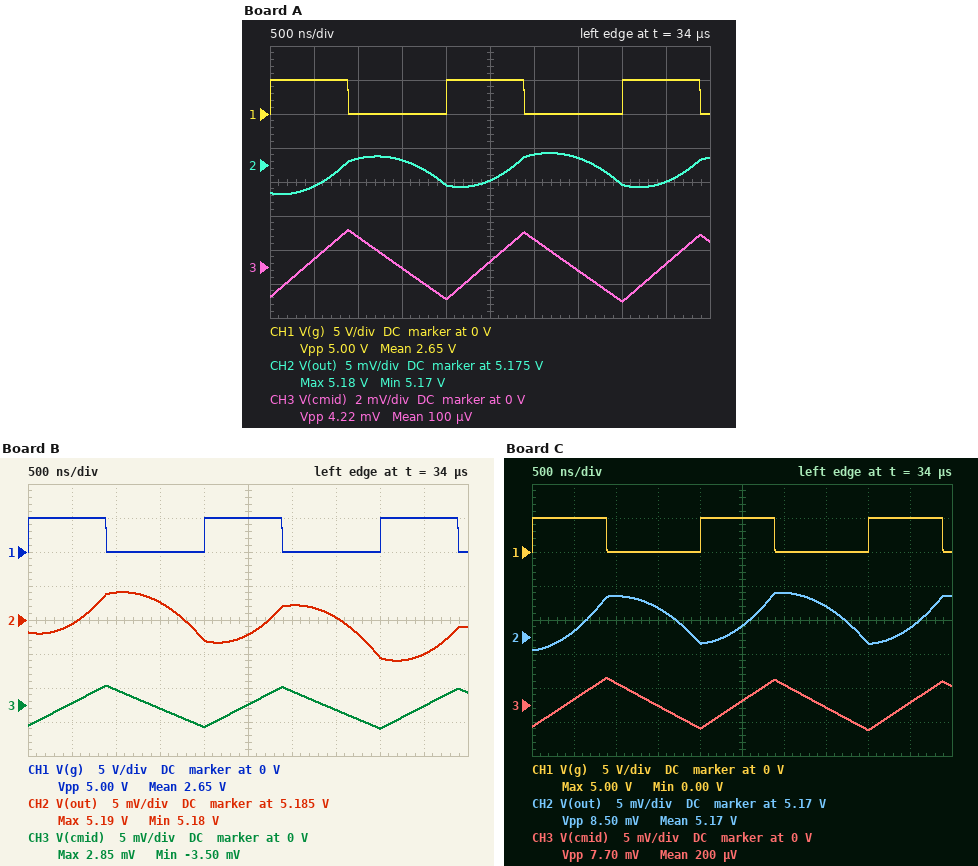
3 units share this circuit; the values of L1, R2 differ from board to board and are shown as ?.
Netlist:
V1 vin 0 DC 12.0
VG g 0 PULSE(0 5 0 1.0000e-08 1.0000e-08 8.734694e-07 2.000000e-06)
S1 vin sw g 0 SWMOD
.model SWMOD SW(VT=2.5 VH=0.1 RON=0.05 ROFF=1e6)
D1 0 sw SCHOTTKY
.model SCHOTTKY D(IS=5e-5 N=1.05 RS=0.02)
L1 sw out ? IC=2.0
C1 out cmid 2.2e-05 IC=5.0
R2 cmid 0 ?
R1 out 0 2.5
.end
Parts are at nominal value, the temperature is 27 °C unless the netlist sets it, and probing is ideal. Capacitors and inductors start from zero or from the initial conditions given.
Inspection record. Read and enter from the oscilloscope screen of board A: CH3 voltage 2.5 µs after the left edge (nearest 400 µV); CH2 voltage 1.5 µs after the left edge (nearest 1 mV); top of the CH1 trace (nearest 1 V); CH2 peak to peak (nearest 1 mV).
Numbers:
400 µV
5.176 V
5 V
6 mV
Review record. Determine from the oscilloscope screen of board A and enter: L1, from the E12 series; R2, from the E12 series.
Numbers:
18 µH
0.012 Ω
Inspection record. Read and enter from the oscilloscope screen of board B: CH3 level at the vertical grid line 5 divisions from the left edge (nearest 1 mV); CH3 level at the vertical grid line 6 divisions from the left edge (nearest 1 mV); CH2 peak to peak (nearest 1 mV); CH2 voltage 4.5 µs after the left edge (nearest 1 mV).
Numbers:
0 V
2 mV
10 mV
5.180 V
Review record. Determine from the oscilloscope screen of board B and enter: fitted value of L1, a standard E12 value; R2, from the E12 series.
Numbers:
15 µH
0.015 Ω
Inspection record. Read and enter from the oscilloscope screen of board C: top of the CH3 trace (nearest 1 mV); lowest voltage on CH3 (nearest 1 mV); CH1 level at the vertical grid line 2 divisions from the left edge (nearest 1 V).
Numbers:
4 mV
-4 mV
0 V
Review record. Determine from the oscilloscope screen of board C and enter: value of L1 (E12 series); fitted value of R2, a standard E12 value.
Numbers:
18 µH
0.022 Ω
